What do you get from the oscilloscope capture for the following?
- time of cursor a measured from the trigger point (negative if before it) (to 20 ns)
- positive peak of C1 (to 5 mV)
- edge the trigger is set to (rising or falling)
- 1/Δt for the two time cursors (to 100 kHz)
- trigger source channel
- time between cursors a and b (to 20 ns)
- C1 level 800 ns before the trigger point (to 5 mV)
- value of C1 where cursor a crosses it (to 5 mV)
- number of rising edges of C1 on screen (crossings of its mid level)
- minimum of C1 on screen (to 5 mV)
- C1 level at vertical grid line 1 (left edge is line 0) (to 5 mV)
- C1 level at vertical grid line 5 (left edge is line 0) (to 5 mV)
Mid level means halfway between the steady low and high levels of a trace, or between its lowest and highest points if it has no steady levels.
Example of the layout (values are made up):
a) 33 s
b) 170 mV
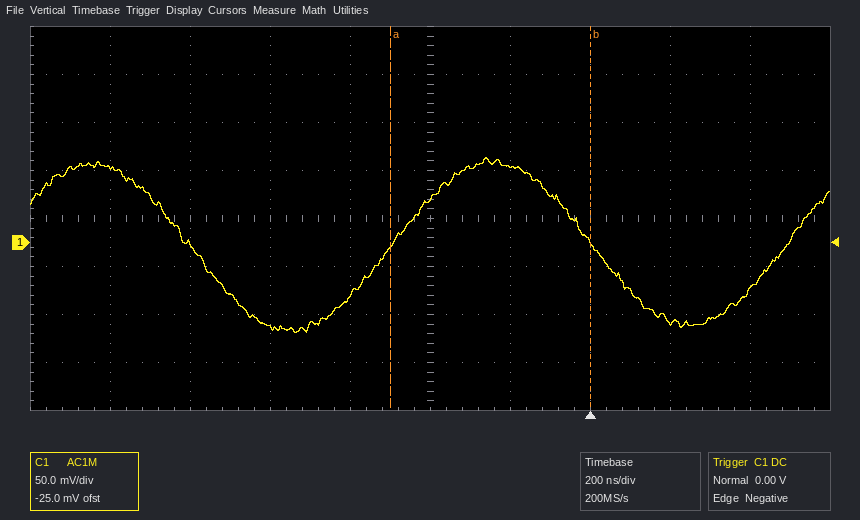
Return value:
a) -500 ns
b) 90 mV
c) falling
d) 2.0 MHz
e) C1
f) 500 ns
g) -90 mV
h) -5 mV
i) 2
j) -95 mV
k) 80 mV
l) 45 mV
